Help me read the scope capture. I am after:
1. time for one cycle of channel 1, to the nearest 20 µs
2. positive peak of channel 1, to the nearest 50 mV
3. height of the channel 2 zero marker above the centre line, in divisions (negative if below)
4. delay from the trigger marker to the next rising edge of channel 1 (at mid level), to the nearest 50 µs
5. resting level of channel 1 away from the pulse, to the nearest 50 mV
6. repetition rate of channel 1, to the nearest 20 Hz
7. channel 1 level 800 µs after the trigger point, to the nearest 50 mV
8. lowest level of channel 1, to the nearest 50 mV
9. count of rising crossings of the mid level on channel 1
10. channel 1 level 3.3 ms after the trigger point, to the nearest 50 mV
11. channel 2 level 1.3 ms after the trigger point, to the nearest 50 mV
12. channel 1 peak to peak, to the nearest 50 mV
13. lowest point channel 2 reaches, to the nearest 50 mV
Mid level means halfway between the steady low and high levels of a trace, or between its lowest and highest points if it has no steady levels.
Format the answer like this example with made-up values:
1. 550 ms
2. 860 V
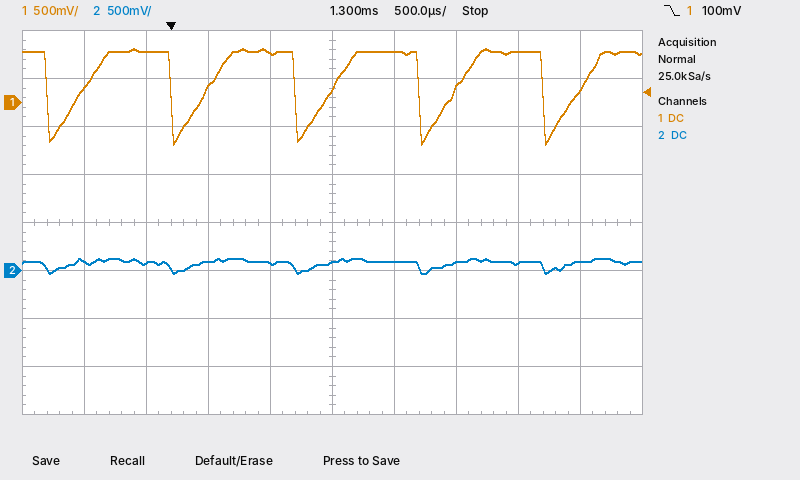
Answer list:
1. 1.00 ms
2. 550 mV
3. -1.0 div
4. 250 µs
5. 550 mV
6. 1.00 kHz
7. 500 mV
8. -450 mV
9. 5
10. 150 mV
11. 100 mV
12. 1.00 V
13. -50 mV
